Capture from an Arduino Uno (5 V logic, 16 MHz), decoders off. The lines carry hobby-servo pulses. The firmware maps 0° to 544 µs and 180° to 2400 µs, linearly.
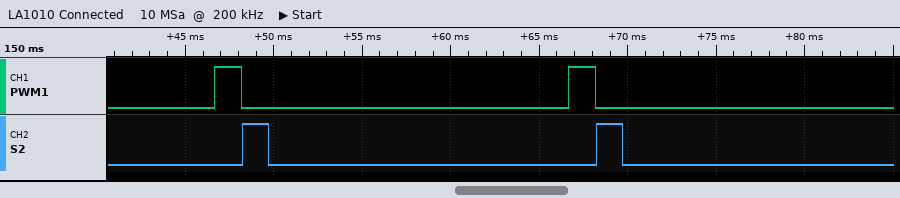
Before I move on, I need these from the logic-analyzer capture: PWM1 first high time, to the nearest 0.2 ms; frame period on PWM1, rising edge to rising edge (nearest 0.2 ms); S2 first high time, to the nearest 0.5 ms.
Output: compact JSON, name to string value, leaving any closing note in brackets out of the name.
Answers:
{"PWM1 first high time, to the nearest 0.2 ms": "1.6 ms", "frame period on PWM1, rising edge to rising edge": "20.0 ms", "S2 first high time, to the nearest 0.5 ms": "1.5 ms"}
